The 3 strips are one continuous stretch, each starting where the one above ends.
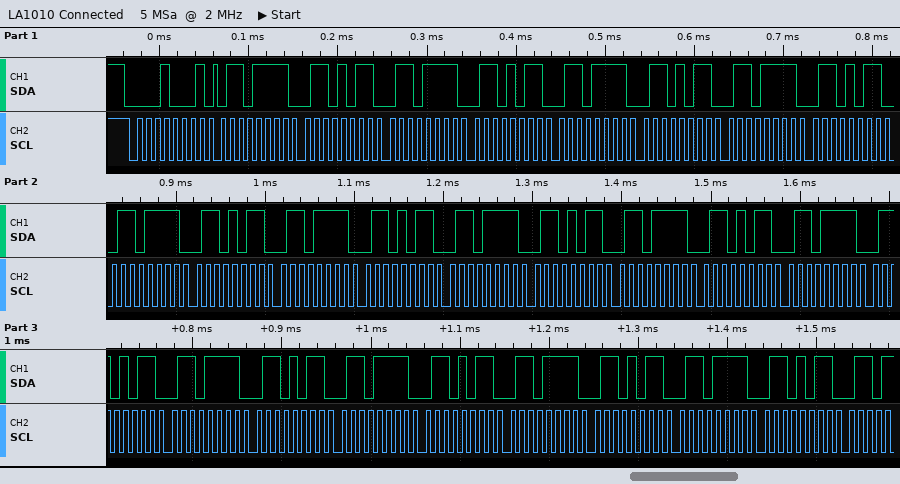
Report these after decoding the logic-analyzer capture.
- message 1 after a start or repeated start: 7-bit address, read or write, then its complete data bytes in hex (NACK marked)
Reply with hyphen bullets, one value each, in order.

- 0x08 read: 6F 6B 6F 6B 6F 6B 6F 6B 6F 6B 6F 6B 6F 6B 6F 6B 6F 6B 6F 6B 6F 6B 6F 6B 6F 6B
